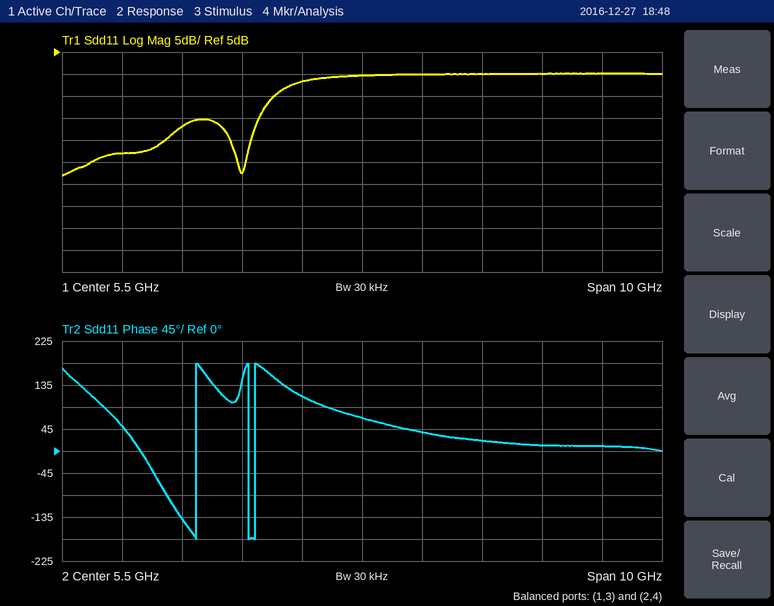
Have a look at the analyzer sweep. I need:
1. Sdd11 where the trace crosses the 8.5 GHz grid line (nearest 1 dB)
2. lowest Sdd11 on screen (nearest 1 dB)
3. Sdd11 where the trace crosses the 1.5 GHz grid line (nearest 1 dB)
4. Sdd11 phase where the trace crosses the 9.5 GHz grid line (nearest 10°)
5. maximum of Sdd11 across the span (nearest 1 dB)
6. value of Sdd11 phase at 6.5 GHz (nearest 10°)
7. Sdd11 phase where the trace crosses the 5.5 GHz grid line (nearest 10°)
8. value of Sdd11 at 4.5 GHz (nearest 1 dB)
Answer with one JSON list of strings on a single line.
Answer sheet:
["0 dB", "-23 dB", "-18 dB", "10°", "0 dB", "40°", "70°", "-2 dB"]
